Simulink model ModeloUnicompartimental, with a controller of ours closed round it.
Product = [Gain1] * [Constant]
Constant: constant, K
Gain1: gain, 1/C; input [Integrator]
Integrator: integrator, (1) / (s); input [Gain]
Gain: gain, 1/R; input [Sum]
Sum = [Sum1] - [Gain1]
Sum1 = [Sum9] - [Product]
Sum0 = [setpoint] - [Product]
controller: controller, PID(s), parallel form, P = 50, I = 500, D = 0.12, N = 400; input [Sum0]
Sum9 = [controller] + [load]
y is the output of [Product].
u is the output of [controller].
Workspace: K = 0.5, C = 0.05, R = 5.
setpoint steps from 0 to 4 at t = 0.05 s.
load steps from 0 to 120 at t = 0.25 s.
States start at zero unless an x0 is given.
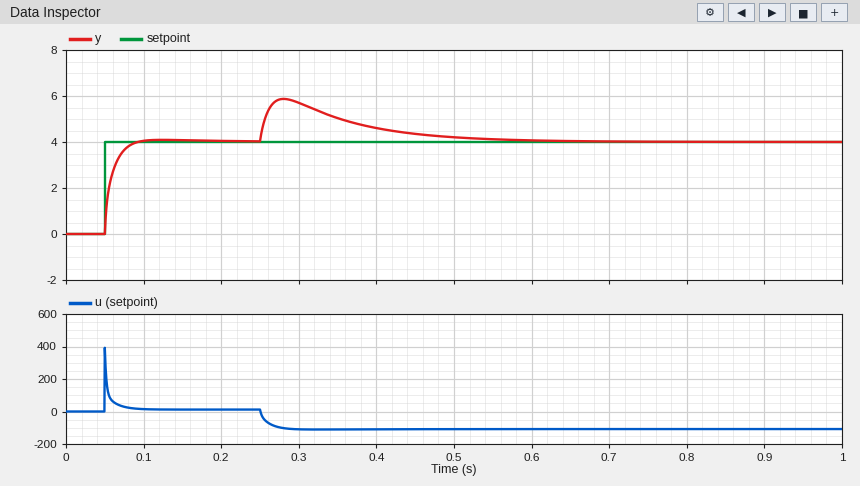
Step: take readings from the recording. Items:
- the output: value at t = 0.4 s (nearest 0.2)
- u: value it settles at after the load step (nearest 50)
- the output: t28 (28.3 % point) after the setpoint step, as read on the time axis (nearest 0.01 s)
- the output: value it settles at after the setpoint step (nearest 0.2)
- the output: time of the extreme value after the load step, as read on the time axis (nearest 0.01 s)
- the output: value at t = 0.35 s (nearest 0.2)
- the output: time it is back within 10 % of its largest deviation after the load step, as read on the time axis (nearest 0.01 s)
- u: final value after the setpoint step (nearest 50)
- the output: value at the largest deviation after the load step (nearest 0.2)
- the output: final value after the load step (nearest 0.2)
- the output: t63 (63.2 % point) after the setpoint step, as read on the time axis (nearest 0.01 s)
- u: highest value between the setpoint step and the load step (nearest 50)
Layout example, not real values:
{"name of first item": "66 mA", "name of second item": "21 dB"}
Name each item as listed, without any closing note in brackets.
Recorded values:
{"the output: value at t = 0.4 s": "4.6", "u: value it settles at after the load step": "-100", "the output: t28 (28.3 % point) after the setpoint step, as read on the time axis": "0.05 s", "the output: value it settles at after the setpoint step": "4.0", "the output: time of the extreme value after the load step, as read on the time axis": "0.28 s", "the output: value at t = 0.35 s": "5.0", "the output: time it is back within 10 % of its largest deviation after the load step, as read on the time axis": "0.51 s", "u: final value after the setpoint step": "0", "the output: value at the largest deviation after the load step": "5.8", "the output: final value after the load step": "4.0", "the output: t63 (63.2 % point) after the setpoint step, as read on the time axis": "0.06 s", "u: highest value between the setpoint step and the load step": "400"}
